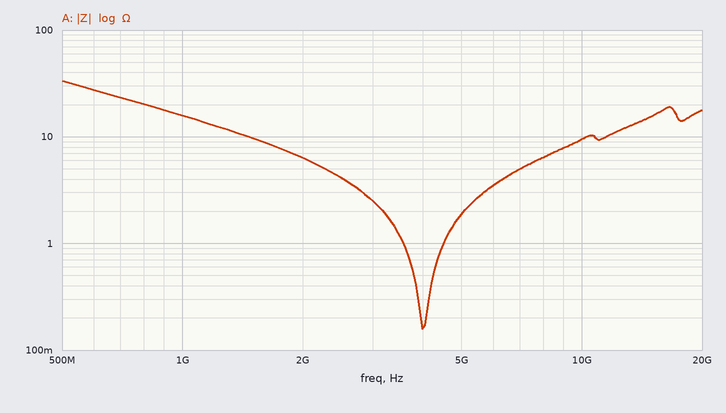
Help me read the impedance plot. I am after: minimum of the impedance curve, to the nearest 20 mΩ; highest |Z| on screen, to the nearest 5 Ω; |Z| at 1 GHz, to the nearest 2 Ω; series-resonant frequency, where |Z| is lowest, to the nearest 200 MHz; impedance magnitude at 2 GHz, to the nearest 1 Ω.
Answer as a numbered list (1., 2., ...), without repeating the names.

1. 160 mΩ
2. 35 Ω
3. 16 Ω
4. 4.0 GHz
5. 6 Ω
